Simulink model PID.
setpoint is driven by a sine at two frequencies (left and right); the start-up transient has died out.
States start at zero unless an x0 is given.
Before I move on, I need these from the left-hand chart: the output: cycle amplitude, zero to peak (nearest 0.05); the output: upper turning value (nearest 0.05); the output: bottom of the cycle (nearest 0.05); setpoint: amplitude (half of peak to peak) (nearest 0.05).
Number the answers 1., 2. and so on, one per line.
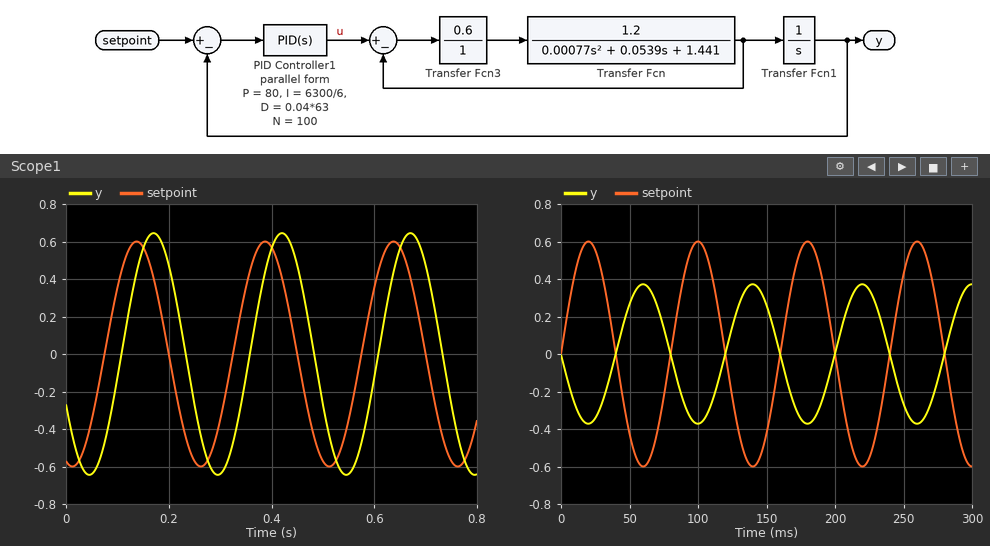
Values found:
1. 0.65
2. 0.65
3. -0.65
4. 0.60
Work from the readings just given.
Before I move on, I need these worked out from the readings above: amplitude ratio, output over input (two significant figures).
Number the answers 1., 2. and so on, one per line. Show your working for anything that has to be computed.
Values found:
1. 0.65 / 0.6 = 1.1
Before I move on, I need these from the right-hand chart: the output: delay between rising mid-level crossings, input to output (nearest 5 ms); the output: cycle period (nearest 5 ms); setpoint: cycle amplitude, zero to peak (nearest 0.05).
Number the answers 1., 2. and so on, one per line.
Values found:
1. 40 ms
2. 80 ms
3. 0.60
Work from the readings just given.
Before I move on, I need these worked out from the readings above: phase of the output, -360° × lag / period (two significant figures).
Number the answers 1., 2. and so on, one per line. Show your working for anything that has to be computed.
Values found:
1. -360 × 40 / 80 = -180°
